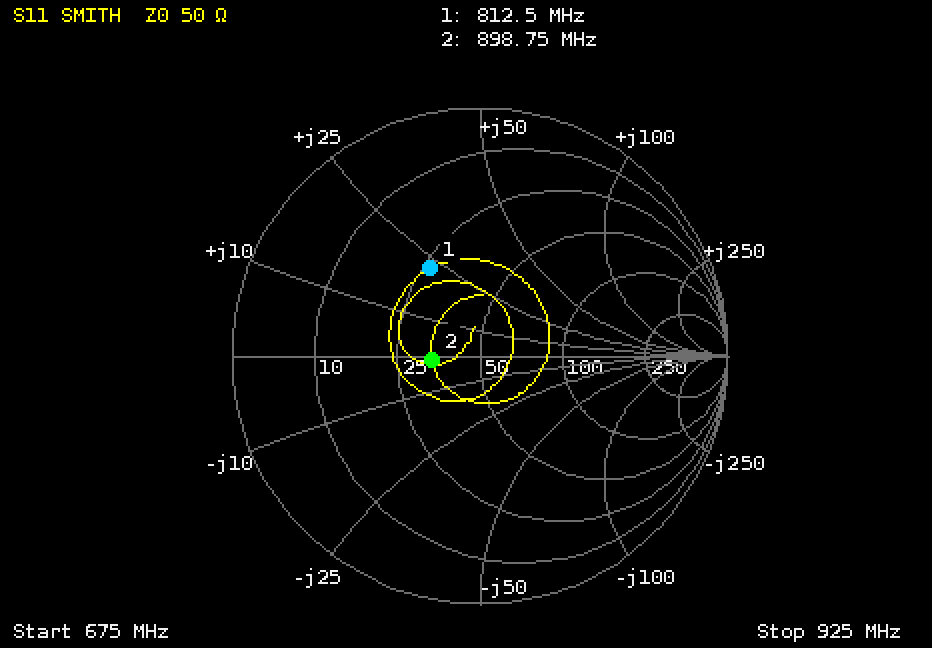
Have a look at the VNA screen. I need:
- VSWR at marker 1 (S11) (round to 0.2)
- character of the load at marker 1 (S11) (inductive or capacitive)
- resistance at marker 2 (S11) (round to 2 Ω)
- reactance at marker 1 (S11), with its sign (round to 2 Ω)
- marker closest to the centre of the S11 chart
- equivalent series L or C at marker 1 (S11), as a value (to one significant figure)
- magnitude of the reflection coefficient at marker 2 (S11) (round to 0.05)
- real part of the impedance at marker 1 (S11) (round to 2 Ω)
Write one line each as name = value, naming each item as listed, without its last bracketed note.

VSWR at marker 1 (S11) = 2.4
character of the load at marker 1 (S11) = inductive
resistance at marker 2 (S11) = 34 Ω
reactance at marker 1 (S11), with its sign = +22 Ω
marker closest to the centre of the S11 chart = marker 2
equivalent series L or C at marker 1 (S11), as a value = 4 nH
magnitude of the reflection coefficient at marker 2 (S11) = 0.20
real part of the impedance at marker 1 (S11) = 26 Ω
